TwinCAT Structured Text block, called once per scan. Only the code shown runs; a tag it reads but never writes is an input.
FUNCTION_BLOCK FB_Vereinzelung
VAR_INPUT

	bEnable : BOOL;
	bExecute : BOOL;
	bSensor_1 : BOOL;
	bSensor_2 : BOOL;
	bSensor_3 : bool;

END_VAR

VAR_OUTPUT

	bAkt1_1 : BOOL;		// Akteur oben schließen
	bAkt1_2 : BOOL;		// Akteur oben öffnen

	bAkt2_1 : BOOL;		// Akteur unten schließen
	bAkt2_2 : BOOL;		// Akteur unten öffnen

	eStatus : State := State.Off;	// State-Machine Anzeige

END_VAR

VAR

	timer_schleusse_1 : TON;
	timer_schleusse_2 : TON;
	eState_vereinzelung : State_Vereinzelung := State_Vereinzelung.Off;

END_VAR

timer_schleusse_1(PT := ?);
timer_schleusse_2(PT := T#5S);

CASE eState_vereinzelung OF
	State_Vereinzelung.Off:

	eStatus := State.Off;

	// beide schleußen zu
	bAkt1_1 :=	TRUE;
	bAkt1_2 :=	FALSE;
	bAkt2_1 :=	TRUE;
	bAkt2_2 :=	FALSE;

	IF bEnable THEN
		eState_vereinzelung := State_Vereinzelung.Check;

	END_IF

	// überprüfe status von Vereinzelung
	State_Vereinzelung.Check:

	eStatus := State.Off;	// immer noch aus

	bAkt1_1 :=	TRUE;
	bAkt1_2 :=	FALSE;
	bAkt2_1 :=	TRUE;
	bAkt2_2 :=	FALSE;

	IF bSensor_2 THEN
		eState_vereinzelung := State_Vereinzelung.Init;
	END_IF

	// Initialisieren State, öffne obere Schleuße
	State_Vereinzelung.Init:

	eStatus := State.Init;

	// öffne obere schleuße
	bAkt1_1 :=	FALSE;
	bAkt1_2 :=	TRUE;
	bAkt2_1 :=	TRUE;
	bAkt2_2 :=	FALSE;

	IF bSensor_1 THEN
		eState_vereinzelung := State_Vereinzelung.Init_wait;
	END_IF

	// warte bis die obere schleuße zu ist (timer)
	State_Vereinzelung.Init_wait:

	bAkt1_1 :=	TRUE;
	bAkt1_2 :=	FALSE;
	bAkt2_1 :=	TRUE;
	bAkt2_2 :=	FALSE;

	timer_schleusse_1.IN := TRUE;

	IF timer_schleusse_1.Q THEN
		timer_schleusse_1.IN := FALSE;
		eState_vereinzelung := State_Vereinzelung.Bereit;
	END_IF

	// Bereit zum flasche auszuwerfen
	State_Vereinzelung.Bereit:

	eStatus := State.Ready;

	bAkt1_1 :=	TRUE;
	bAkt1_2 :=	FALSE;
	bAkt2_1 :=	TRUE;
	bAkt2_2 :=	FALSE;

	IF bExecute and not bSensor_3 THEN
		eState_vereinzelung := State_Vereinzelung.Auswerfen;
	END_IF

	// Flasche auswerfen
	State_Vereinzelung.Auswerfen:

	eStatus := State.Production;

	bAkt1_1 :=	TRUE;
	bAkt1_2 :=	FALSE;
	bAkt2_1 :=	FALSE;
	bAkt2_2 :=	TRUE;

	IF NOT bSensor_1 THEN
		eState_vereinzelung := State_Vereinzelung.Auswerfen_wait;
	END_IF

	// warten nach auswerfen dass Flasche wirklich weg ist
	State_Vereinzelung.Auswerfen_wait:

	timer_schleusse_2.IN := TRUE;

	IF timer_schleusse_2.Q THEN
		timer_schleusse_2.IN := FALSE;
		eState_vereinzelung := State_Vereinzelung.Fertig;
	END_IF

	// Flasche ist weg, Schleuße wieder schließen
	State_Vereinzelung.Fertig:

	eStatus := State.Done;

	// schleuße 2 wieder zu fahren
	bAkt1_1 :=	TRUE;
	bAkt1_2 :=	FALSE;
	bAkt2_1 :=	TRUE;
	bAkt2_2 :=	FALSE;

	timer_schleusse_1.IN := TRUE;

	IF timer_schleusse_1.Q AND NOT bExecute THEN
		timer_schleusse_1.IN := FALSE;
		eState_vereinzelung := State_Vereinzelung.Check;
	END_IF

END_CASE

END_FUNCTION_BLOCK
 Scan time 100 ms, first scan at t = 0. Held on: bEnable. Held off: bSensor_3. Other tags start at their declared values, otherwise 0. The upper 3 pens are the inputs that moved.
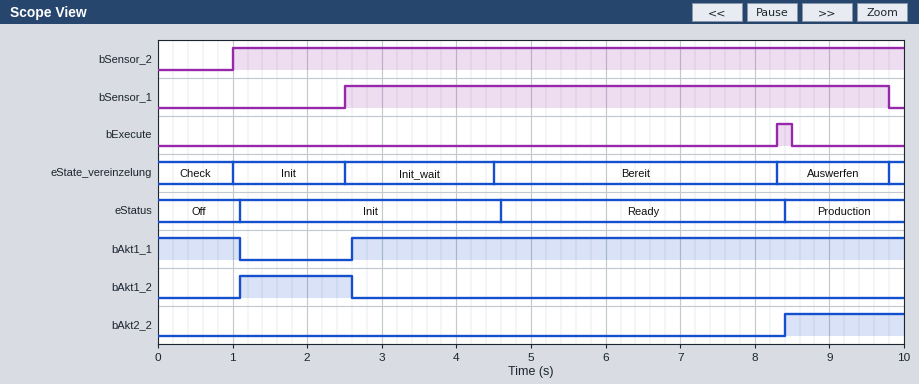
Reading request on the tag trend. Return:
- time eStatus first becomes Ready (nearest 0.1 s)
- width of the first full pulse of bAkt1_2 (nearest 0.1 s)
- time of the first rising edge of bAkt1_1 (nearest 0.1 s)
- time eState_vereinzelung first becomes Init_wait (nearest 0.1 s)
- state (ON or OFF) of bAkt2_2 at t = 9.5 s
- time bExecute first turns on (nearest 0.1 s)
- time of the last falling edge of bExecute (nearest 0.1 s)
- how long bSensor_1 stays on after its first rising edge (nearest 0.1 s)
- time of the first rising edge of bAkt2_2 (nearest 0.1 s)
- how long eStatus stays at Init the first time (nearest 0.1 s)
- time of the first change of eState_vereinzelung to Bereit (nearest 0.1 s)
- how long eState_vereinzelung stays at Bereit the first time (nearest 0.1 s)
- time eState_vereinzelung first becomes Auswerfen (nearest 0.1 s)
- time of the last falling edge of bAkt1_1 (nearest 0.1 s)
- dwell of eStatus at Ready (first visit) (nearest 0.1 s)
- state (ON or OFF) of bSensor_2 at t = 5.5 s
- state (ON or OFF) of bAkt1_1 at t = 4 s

4.6 s
1.5 s
2.6 s
2.5 s
ON
8.3 s
8.5 s
7.3 s
8.4 s
3.5 s
4.5 s
3.8 s
8.3 s
1.1 s
3.8 s
ON
ON
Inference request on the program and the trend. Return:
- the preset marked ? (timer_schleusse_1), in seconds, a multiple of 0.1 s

1.8 s
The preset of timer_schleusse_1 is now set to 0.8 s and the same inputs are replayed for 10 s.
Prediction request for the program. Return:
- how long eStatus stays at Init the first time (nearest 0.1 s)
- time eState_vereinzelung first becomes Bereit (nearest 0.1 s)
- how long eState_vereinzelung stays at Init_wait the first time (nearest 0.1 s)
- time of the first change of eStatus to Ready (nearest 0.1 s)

2.5 s
3.5 s
1.0 s
3.6 s
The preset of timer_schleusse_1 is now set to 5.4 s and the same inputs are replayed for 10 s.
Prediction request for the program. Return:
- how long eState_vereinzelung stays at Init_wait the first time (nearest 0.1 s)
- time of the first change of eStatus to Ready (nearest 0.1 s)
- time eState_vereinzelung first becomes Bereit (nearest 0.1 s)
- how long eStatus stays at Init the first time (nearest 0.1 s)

5.6 s
8.2 s
8.1 s
7.1 s
